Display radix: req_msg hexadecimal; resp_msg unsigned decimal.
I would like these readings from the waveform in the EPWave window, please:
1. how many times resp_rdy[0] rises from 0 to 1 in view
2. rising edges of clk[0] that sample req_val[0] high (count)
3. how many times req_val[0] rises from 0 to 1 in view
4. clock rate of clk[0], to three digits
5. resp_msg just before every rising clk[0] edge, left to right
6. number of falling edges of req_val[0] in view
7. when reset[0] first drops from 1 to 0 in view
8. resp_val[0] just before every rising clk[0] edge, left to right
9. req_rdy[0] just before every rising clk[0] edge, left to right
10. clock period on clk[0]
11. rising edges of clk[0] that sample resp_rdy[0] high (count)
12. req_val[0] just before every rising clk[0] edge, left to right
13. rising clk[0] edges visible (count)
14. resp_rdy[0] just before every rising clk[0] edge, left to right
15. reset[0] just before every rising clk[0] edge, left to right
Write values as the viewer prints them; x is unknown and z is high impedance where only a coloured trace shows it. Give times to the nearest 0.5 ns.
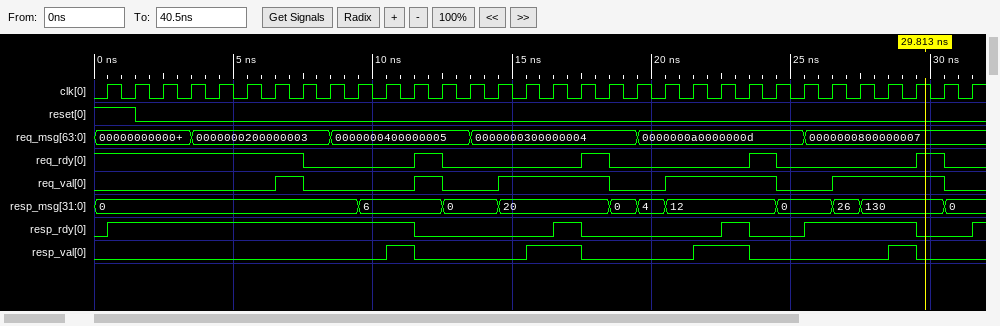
5
14
5
1.00 GHz
0, 0, 0, 0, 0, 0, 0, 0, 0, 0, 6, 6, 6, 0, 0, 20, 20, 20, 20, 0, 4, 12, 12, 12, 12, 0, 0, 26, 130, 130, 130, 0
5
1.5 ns
0 0 0 0 0 0 0 0 0 0 0 1 0 0 0 0 1 1 0 0 0 0 1 1 0 0 0 0 0 1 0 0
1 1 1 1 1 1 1 1 0 0 0 0 1 0 0 0 0 0 1 0 0 0 0 0 1 0 0 0 0 0 1 0
1 ns
17
0 0 0 0 0 0 0 1 0 0 0 0 1 0 0 1 1 1 1 0 0 1 1 1 1 0 0 1 1 1 1 0
32
0 1 1 1 1 1 1 1 1 1 1 1 0 0 0 0 0 1 0 0 0 0 0 1 0 0 1 1 1 1 0 0
1 1 0 0 0 0 0 0 0 0 0 0 0 0 0 0 0 0 0 0 0 0 0 0 0 0 0 0 0 0 0 0
